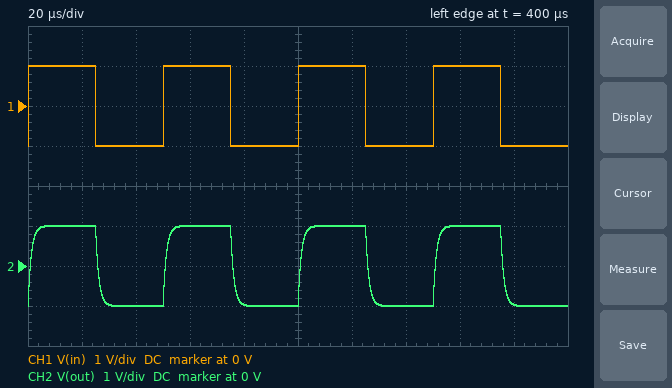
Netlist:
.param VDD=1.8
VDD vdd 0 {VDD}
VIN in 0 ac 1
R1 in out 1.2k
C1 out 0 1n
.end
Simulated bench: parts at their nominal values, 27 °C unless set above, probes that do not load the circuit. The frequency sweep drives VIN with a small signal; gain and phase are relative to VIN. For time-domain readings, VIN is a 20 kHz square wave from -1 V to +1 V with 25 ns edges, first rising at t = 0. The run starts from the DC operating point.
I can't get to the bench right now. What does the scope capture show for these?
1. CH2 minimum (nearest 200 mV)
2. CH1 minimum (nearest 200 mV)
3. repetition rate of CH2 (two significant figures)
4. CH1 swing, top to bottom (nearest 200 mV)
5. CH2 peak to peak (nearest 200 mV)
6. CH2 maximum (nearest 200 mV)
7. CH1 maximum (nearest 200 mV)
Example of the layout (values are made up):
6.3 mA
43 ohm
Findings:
-1.0 V
-1.0 V
20 kHz
2.0 V
2.0 V
1.0 V
1.0 V
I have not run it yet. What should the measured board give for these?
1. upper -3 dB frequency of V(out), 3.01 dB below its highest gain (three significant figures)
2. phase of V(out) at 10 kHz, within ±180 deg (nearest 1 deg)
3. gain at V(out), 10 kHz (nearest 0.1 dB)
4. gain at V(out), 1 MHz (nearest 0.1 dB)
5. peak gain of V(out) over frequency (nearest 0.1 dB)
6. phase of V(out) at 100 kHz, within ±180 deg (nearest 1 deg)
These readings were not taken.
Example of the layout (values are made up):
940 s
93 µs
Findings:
133 kHz
-4 deg
0 dB
-17.6 dB
0 dB
-37 deg
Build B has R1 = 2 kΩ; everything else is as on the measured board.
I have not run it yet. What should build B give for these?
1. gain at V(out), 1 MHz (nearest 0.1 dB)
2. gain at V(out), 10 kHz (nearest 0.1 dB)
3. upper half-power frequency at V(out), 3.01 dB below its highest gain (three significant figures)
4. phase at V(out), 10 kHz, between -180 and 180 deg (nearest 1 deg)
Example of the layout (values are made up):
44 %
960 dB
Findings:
-22.0 dB
-0.1 dB
79.6 kHz
-7 deg
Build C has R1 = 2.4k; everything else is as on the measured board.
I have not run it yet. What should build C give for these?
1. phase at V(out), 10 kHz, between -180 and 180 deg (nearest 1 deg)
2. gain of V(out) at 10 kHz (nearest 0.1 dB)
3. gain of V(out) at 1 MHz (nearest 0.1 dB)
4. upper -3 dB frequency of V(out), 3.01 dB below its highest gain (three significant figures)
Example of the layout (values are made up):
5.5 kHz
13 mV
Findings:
-9 deg
-0.1 dB
-23.6 dB
66.3 kHz
